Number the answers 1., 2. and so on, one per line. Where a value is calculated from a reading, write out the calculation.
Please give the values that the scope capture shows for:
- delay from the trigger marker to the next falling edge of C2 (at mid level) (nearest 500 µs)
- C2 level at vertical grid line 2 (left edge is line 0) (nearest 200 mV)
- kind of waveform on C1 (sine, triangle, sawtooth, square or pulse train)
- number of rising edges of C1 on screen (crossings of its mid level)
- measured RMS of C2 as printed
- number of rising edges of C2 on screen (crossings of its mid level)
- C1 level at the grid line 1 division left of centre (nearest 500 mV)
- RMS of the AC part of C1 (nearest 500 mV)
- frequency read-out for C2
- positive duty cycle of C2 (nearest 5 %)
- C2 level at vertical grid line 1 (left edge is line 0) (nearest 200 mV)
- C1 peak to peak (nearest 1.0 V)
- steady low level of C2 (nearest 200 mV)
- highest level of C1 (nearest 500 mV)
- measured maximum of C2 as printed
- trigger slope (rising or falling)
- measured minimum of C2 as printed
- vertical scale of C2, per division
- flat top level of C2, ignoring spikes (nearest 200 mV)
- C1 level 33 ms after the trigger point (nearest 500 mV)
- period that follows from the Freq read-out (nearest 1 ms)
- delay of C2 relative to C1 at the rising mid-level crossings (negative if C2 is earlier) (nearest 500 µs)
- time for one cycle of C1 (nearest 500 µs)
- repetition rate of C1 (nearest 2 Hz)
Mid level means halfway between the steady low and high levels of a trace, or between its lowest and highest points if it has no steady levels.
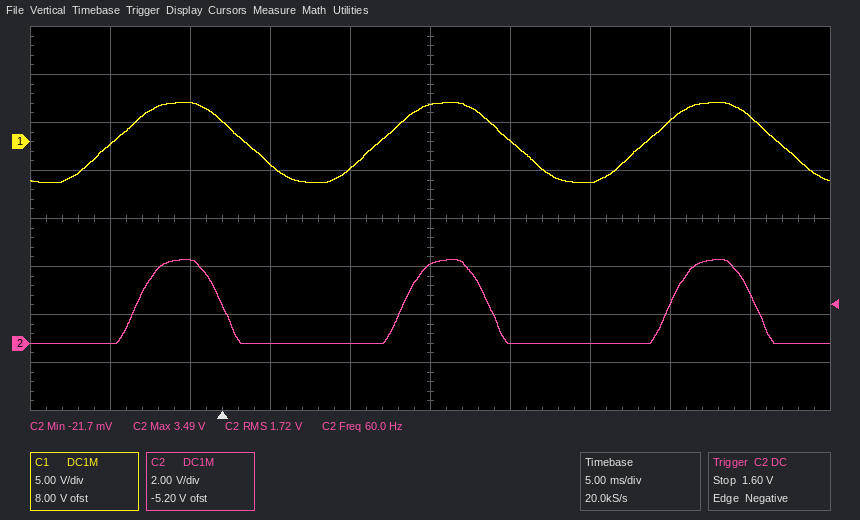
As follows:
1. 16.5 ms
2. 3.4 V
3. sine
4. 3
5. 1.72 V
6. 3
7. -3.0 V
8. 8.0 V / (2√2) ≈ 2.83 V, so 3.0 V to the nearest 500 mV
9. 60.0 Hz
10. 30 %
11. 0.0 V
12. 8.0 V
13. 0.0 V
14. 4.0 V
15. 3.49 V
16. falling
17. -21.7 mV
18. 2 V
19. 3.4 V
20. 2.5 V
21. 1 / 60.0 Hz ≈ 17 ms
22. +1.5 ms
23. 16.5 ms
24. 1 / 16.5 ms ≈ 60.6 Hz, so 60 Hz to the nearest 2 Hz
